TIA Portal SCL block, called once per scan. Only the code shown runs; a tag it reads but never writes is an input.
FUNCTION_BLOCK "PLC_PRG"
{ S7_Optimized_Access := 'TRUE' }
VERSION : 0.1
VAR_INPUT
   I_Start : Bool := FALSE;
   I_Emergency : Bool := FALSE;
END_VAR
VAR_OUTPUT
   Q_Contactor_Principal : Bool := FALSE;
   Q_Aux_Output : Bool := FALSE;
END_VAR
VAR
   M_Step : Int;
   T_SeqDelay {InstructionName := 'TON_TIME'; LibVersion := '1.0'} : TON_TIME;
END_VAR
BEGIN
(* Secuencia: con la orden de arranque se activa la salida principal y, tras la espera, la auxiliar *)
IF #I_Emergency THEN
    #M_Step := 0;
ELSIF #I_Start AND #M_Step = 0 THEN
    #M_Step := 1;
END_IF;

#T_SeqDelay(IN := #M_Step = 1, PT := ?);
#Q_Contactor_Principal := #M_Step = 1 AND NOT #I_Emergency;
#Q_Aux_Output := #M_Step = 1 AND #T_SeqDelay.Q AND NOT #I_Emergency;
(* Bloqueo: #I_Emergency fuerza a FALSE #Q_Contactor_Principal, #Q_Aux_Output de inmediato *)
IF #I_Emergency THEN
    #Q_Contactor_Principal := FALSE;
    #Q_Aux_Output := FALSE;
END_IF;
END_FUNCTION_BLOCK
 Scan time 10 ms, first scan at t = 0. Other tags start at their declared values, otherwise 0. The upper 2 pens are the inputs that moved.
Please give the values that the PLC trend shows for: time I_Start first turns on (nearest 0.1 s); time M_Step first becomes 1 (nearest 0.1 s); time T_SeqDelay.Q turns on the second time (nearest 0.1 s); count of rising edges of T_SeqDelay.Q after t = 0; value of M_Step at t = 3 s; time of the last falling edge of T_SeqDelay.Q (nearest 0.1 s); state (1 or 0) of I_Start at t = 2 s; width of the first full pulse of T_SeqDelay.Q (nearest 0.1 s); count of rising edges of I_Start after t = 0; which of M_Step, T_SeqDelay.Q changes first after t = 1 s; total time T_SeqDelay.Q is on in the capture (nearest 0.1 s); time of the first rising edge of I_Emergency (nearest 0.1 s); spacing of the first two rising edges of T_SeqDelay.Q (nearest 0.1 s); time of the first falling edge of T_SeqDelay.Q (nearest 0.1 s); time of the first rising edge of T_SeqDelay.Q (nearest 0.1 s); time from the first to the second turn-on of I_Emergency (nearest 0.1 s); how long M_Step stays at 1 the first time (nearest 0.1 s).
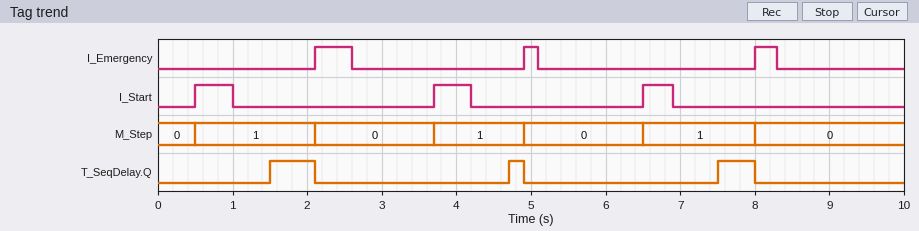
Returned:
0.5 s
0.5 s
4.7 s
3
0
8.0 s
0
0.6 s
3
T_SeqDelay.Q
1.3 s
2.1 s
3.2 s
2.1 s
1.5 s
2.8 s
1.6 s
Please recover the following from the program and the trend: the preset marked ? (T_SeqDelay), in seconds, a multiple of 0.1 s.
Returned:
1.0 s
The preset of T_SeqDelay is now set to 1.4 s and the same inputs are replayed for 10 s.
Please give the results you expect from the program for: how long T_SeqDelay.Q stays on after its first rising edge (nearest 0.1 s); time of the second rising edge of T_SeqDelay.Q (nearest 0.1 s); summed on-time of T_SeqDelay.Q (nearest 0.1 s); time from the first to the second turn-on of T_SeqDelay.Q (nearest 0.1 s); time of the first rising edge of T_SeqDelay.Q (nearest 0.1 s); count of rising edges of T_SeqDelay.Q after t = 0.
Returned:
0.2 s
7.9 s
0.3 s
6.0 s
1.9 s
2
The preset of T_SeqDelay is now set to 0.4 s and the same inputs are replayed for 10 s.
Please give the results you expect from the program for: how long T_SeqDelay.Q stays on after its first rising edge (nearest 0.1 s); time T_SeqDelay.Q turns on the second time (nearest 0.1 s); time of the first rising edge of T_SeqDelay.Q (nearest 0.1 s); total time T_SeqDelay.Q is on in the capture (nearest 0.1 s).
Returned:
1.2 s
4.1 s
0.9 s
3.1 s
